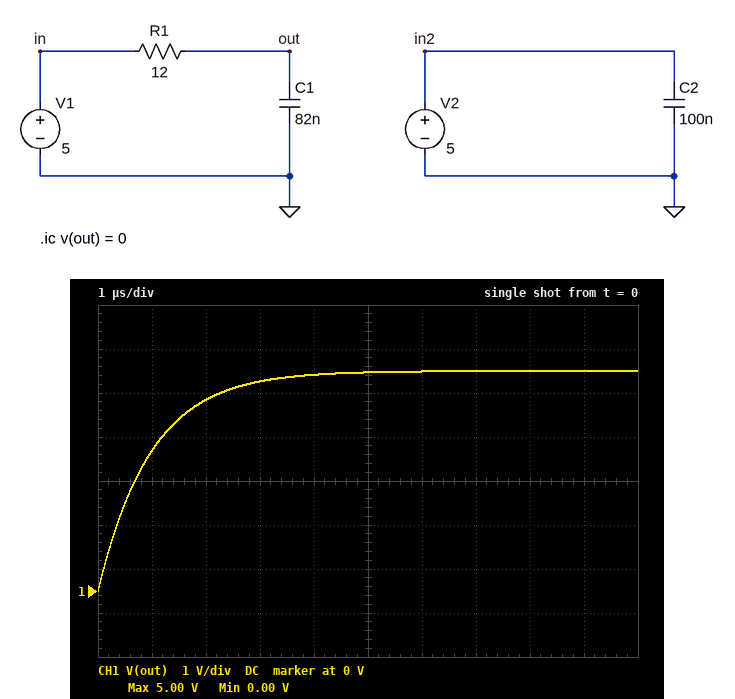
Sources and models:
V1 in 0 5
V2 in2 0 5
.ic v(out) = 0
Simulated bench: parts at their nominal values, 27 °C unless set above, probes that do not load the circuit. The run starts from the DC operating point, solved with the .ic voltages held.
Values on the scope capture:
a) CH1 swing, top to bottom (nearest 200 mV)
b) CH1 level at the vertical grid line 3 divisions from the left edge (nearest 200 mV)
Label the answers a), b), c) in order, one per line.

a) 5.0 V
b) 4.8 V
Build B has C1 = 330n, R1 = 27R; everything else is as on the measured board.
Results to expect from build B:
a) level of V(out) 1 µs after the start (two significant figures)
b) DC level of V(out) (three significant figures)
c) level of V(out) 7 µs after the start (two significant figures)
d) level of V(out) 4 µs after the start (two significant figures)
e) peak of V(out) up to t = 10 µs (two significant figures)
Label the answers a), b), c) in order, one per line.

a) 530 mV
b) 5.00 V
c) 2.7 V
d) 1.8 V
e) 3.4 V
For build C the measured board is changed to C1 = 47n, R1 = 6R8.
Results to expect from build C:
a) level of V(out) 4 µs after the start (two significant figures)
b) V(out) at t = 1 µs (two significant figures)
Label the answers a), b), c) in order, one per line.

a) 5.0 V
b) 4.8 V
